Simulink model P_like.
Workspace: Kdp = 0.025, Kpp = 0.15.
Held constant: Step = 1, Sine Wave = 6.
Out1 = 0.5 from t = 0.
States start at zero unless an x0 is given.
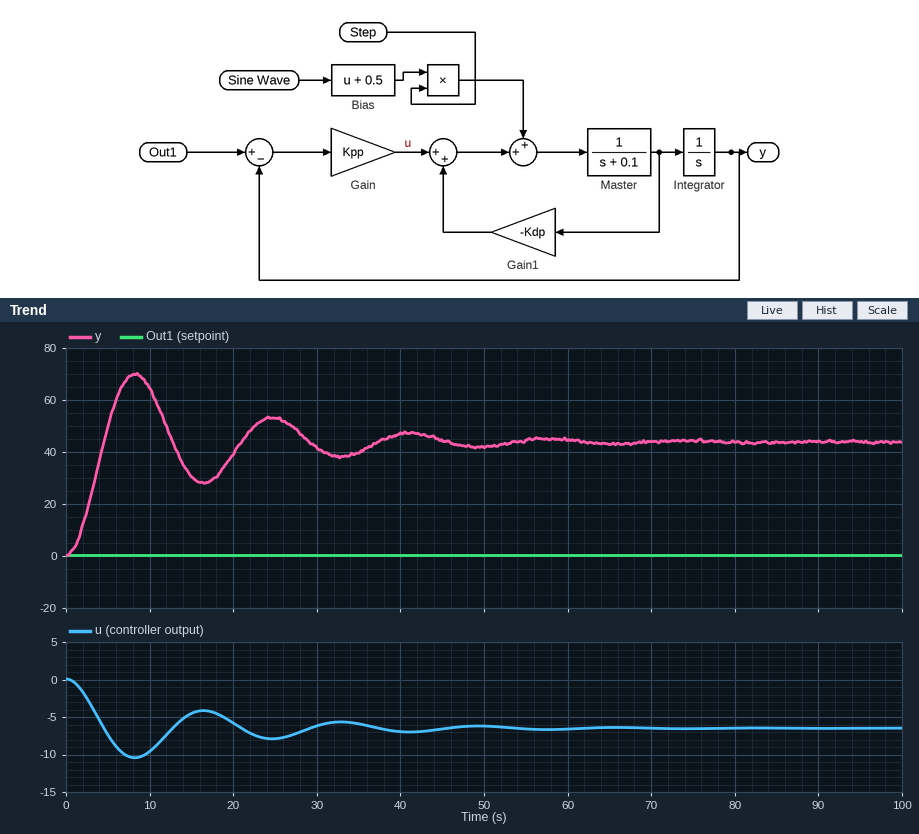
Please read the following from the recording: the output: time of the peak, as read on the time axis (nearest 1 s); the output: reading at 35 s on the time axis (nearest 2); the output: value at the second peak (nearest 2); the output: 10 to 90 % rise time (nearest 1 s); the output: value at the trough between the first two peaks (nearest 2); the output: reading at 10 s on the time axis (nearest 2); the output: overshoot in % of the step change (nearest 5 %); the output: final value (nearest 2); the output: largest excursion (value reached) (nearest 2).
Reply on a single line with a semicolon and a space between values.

8 s; 40; 54; 3 s; 28; 64; 60 %; 44; 70
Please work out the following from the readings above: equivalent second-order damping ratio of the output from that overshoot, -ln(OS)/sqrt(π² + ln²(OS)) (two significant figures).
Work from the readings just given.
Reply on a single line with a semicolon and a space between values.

0.16
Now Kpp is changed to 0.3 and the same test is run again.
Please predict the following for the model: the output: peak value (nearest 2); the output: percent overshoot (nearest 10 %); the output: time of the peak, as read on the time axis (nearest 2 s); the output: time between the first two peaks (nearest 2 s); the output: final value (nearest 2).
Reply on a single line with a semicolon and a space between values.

38; 70 %; 6 s; 12 s; 22
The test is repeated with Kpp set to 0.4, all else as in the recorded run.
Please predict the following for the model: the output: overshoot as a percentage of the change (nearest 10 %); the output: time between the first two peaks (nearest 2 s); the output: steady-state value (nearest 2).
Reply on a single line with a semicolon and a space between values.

70 %; 10 s; 16
